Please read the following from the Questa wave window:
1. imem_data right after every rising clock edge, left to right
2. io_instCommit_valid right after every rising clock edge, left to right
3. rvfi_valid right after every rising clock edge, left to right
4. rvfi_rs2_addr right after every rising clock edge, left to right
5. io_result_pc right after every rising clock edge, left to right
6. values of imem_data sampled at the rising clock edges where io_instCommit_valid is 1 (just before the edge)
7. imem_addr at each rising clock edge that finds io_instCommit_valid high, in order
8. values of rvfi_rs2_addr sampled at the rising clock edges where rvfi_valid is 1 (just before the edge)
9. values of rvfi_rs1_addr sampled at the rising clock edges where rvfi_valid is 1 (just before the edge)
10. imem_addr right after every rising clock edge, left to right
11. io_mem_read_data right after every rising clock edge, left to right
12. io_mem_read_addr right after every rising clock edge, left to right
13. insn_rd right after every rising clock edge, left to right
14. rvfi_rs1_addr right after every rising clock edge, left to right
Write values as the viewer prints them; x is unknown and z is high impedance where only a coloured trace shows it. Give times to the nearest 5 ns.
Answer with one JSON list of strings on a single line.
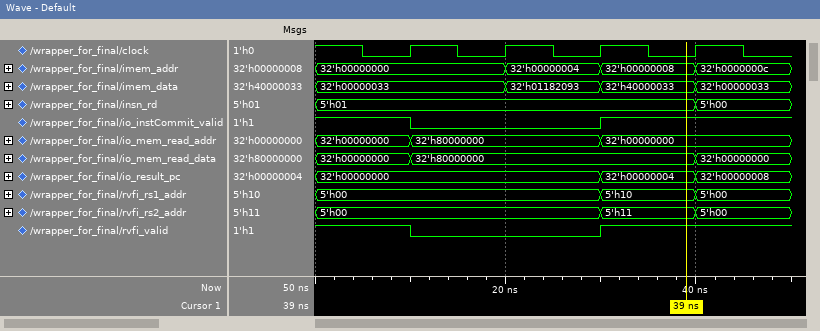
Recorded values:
["32'h00000033, 32'h01182093, 32'h40000033, 32'h00000033", "0 0 1 1", "0 0 1 1", "5'h00, 5'h00, 5'h11, 5'h00", "32'h00000000, 32'h00000000, 32'h00000004, 32'h00000008", "32'h00000033, 32'h40000033", "32'h00000000, 32'h00000008", "5'h00, 5'h11", "5'h00, 5'h10", "32'h00000000, 32'h00000004, 32'h00000008, 32'h0000000c", "32'h80000000, 32'h80000000, 32'h80000000, 32'h00000000", "32'h80000000, 32'h80000000, 32'h00000000, 32'h00000000", "5'h01, 5'h01, 5'h01, 5'h00", "5'h00, 5'h00, 5'h10, 5'h00"]
